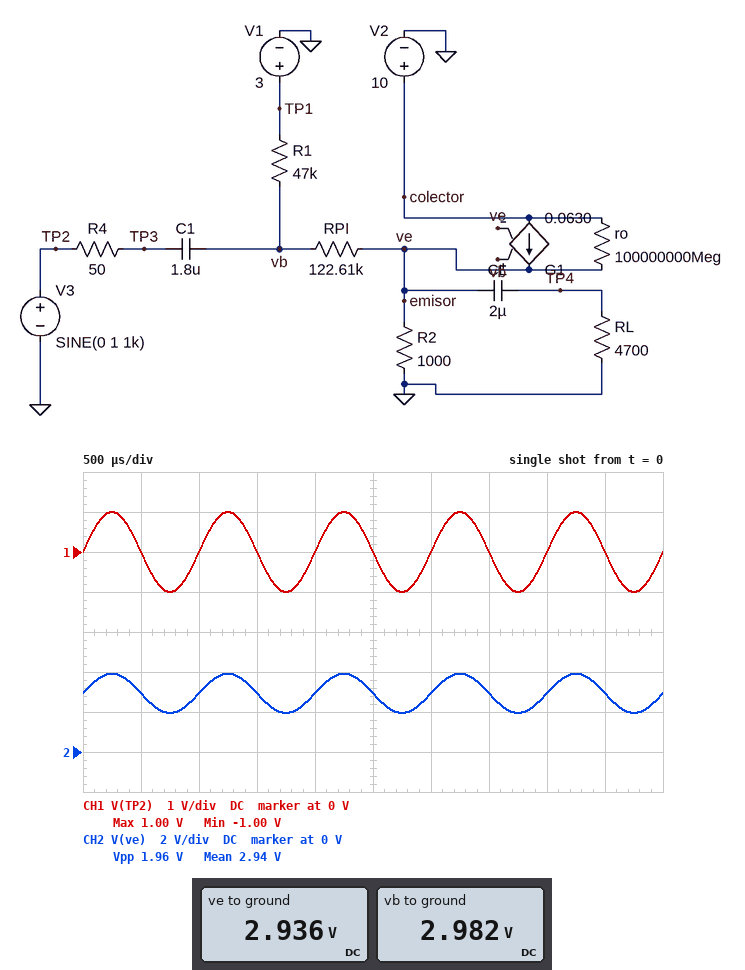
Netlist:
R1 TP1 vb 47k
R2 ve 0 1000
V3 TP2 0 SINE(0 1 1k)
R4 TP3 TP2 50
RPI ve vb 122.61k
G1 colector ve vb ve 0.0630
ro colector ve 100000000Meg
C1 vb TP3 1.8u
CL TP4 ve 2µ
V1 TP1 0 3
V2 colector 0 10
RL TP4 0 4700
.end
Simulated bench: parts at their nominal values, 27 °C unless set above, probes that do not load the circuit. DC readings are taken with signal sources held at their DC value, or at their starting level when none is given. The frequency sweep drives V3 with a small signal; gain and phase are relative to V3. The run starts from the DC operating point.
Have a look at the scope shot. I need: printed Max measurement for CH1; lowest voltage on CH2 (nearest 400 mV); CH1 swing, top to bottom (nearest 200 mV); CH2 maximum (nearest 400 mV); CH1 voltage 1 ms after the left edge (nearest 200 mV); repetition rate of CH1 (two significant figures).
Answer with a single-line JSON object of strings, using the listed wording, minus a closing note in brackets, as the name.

{"printed Max measurement for CH1": "1.00 V", "lowest voltage on CH2": "2.0 V", "CH1 swing, top to bottom": "2.0 V", "CH2 maximum": "4.0 V", "CH1 voltage 1 ms after the left edge": "0 V", "repetition rate of CH1": "1.0 kHz"}
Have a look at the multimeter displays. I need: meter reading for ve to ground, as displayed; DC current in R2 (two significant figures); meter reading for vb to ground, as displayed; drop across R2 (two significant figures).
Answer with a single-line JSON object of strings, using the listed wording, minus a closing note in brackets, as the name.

{"meter reading for ve to ground, as displayed": "2.936 V", "DC current in R2": "2.9 mA", "meter reading for vb to ground, as displayed": "2.982 V", "drop across R2": "2.9 V"}
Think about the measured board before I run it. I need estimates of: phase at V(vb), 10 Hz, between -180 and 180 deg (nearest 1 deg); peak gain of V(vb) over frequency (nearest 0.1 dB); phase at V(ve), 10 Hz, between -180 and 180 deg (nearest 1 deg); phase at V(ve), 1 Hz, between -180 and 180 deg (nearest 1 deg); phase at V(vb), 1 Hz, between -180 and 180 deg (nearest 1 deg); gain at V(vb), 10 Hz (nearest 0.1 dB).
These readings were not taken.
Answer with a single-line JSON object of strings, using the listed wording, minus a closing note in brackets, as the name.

{"phase at V(vb), 10 Hz, between -180 and 180 deg": "11 deg", "peak gain of V(vb) over frequency": "0 dB", "phase at V(ve), 10 Hz, between -180 and 180 deg": "11 deg", "phase at V(ve), 1 Hz, between -180 and 180 deg": "62 deg", "phase at V(vb), 1 Hz, between -180 and 180 deg": "62 deg", "gain at V(vb), 10 Hz": "-0.2 dB"}
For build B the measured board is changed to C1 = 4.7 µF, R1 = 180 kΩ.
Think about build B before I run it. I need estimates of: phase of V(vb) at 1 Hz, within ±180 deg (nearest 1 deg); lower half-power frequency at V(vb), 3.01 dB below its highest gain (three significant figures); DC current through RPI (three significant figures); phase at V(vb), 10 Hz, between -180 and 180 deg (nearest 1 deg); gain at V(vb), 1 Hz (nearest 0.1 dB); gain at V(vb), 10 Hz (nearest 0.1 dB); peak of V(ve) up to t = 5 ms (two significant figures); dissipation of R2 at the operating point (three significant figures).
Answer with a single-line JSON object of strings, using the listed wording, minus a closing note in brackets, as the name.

{"phase of V(vb) at 1 Hz, within ±180 deg": "11 deg", "lower half-power frequency at V(vb), 3.01 dB below its highest gain": "192 mHz", "DC current through RPI": "374 nA", "phase at V(vb), 10 Hz, between -180 and 180 deg": "1 deg", "gain at V(vb), 1 Hz": "-0.2 dB", "gain at V(vb), 10 Hz": "0 dB", "peak of V(ve) up to t = 5 ms": "3.9 V", "dissipation of R2 at the operating point": "8.33 mW"}
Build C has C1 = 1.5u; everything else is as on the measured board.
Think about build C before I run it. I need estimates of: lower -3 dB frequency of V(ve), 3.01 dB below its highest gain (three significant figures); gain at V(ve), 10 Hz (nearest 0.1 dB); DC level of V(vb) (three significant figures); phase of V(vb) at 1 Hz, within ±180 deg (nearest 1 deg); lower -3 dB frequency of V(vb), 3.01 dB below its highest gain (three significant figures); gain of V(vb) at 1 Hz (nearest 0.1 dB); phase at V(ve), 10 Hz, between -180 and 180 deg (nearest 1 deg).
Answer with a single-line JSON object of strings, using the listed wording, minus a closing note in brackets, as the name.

{"lower -3 dB frequency of V(ve), 3.01 dB below its highest gain": "2.25 Hz", "gain at V(ve), 10 Hz": "-0.4 dB", "DC level of V(vb)": "2.98 V", "phase of V(vb) at 1 Hz, within ±180 deg": "66 deg", "lower -3 dB frequency of V(vb), 3.01 dB below its highest gain": "2.27 Hz", "gain of V(vb) at 1 Hz": "-7.9 dB", "phase at V(ve), 10 Hz, between -180 and 180 deg": "13 deg"}
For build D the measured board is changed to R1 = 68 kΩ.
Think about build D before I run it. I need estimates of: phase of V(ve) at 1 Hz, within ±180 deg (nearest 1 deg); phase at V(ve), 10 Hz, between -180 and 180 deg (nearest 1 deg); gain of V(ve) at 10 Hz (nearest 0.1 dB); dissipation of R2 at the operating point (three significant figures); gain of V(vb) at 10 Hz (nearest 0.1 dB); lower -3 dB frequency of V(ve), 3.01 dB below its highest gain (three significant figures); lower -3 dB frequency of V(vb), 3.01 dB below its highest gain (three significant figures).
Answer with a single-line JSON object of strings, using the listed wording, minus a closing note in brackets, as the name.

{"phase of V(ve) at 1 Hz, within ±180 deg": "53 deg", "phase at V(ve), 10 Hz, between -180 and 180 deg": "7 deg", "gain of V(ve) at 10 Hz": "-0.2 dB", "dissipation of R2 at the operating point": "8.57 mW", "gain of V(vb) at 10 Hz": "-0.1 dB", "lower -3 dB frequency of V(ve), 3.01 dB below its highest gain": "1.30 Hz", "lower -3 dB frequency of V(vb), 3.01 dB below its highest gain": "1.31 Hz"}
